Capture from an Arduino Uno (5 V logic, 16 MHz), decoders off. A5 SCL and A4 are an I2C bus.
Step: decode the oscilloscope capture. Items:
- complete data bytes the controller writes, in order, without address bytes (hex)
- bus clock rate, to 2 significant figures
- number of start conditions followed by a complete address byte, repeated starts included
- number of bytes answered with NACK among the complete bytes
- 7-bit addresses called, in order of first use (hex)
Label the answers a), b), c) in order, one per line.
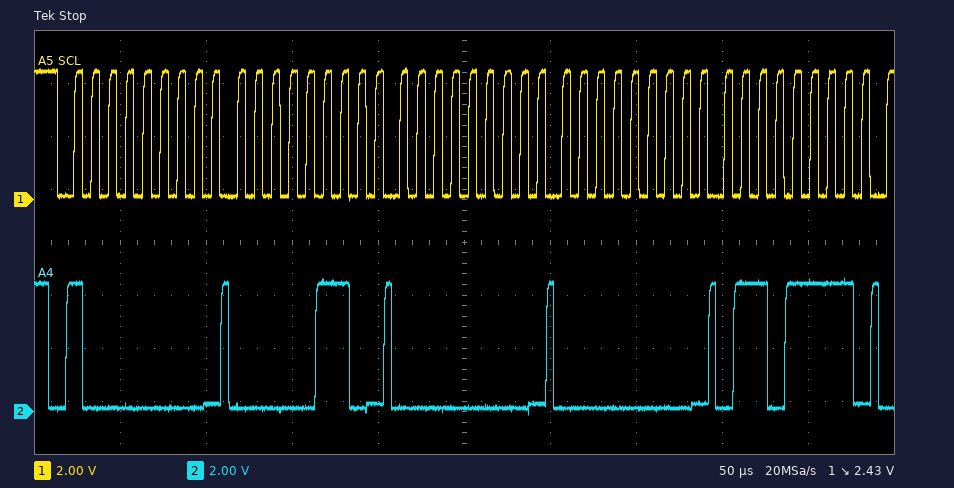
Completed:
a) 06 00 00 6F
b) 100 kHz
c) 1
d) 0
e) 0x40
